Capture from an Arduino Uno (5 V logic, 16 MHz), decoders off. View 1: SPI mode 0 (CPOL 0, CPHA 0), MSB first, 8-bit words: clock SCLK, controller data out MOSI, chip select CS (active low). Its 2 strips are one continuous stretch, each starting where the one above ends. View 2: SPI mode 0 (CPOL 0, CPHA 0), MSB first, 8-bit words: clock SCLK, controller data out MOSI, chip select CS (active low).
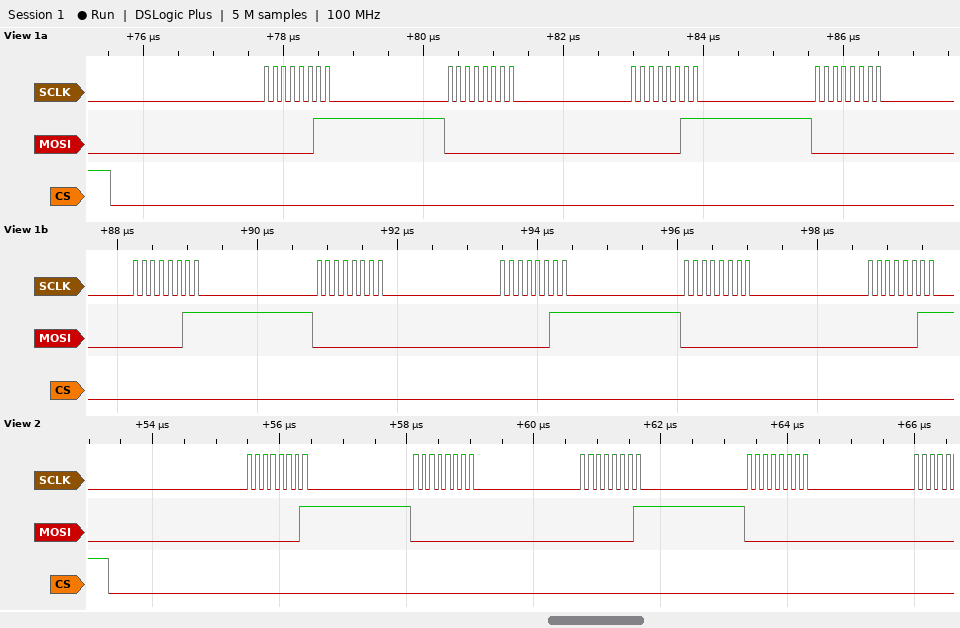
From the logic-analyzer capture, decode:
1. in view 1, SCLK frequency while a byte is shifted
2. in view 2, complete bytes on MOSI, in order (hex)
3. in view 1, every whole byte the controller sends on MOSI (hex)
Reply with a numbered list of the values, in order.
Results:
1. 8 MHz
2. 01 00 01 00
3. 0x03 0x00 0x03 0x00 0x03 0x00 0x03 0x00 0x03
